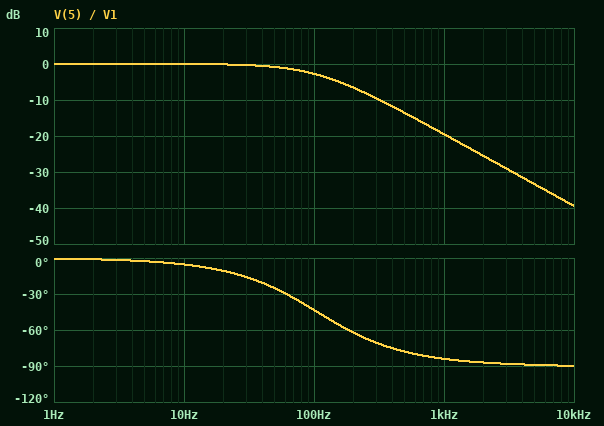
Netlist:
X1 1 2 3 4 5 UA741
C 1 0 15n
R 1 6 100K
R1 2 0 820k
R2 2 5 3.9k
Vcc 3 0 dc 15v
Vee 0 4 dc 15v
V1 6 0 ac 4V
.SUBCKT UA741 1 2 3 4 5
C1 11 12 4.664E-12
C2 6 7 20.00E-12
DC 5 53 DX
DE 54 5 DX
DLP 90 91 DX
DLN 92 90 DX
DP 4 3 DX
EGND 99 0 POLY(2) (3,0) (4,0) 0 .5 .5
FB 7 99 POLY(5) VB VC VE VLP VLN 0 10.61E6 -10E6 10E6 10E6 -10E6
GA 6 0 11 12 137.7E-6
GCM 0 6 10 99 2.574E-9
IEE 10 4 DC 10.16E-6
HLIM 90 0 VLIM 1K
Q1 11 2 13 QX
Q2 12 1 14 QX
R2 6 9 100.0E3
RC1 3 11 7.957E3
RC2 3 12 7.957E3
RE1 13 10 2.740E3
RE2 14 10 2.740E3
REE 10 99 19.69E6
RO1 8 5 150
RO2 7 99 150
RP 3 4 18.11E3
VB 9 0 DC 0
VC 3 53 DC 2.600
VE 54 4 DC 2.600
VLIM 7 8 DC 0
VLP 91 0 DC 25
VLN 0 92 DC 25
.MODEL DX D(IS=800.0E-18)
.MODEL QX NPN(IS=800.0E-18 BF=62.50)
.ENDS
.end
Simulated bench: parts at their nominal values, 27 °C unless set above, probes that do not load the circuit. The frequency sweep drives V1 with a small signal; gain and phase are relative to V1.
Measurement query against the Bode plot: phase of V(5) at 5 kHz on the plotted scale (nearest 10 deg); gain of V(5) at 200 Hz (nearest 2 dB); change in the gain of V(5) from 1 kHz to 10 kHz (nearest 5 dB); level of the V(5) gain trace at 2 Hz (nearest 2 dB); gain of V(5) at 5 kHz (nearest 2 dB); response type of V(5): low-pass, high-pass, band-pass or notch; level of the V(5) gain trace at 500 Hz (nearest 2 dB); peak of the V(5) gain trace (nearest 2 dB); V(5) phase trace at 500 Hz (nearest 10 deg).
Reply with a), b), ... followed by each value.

a) -90 deg
b) -6 dB
c) -20 dB
d) 0 dB
e) -34 dB
f) low-pass
g) -14 dB
h) 0 dB
i) -80 deg
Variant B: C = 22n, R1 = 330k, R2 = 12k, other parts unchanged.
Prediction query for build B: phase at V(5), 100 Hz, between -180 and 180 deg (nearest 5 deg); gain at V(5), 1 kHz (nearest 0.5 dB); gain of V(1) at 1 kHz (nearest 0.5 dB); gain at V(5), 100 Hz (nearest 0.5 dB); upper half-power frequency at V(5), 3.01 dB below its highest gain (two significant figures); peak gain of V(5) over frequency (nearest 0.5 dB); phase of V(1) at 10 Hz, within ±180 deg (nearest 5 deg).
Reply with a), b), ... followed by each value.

a) -55 deg
b) -22.5 dB
c) -23.0 dB
d) -4.5 dB
e) 72 Hz
f) 0.5 dB
g) -10 deg
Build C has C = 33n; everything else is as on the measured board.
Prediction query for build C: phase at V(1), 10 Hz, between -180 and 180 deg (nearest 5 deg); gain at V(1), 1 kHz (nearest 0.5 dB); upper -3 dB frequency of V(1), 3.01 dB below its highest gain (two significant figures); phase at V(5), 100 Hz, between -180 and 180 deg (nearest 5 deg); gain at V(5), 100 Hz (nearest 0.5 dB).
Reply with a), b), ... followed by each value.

a) -10 deg
b) -26.5 dB
c) 48 Hz
d) -65 deg
e) -7.0 dB
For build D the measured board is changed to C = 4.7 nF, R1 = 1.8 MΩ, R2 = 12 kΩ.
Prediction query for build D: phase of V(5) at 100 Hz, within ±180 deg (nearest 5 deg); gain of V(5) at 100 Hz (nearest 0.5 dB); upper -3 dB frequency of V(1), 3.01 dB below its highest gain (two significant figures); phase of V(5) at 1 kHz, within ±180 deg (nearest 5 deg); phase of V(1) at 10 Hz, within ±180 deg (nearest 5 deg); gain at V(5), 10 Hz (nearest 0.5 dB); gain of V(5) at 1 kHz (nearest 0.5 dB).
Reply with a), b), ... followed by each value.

a) -15 deg
b) -0.5 dB
c) 340 Hz
d) -70 deg
e) 0 deg
f) 0 dB
g) -10.0 dB
